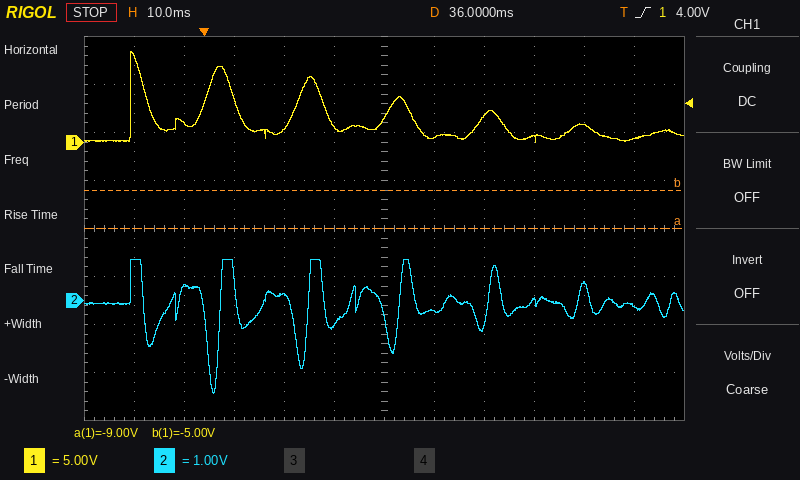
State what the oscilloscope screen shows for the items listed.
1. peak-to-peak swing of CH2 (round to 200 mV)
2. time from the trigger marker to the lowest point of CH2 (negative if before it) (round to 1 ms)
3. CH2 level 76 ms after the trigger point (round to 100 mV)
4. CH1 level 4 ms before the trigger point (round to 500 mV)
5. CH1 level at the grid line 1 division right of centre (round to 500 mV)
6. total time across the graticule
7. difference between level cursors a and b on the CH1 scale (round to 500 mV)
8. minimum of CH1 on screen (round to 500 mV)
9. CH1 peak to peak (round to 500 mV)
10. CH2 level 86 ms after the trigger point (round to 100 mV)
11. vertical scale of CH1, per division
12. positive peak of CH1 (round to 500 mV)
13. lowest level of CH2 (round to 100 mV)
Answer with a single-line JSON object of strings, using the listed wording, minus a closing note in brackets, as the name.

{"peak-to-peak swing of CH2": "2.8 V", "time from the trigger marker to the lowest point of CH2 (negative if before it)": "+2 ms", "CH2 level 76 ms after the trigger point": "300 mV", "CH1 level 4 ms before the trigger point": "2.0 V", "CH1 level at the grid line 1 division right of centre": "500 mV", "total time across the graticule": "120 ms", "difference between level cursors a and b on the CH1 scale": "4.0 V", "minimum of CH1 on screen": "0.0 V", "CH1 peak to peak": "9.5 V", "CH2 level 86 ms after the trigger point": "-100 mV", "vertical scale of CH1, per division": "5 V", "positive peak of CH1": "9.5 V", "lowest level of CH2": "-1.9 V"}
